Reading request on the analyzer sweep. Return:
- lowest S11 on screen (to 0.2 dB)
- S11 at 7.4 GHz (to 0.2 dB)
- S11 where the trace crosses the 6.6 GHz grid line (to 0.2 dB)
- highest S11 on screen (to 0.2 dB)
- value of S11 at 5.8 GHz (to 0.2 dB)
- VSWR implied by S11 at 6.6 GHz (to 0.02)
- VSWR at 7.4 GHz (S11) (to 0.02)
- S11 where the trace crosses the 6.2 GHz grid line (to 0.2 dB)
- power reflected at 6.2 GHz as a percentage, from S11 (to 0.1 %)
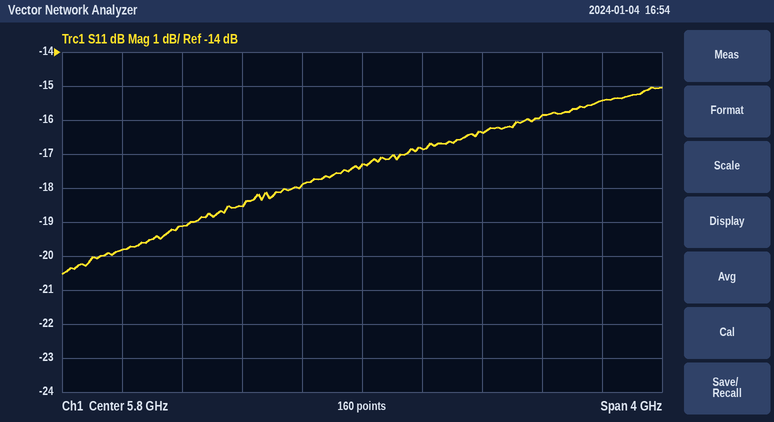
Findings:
-20.6 dB
-15.4 dB
-16.4 dB
-15.0 dB
-17.4 dB
1.36
1.40
-16.8 dB
2.1 %
